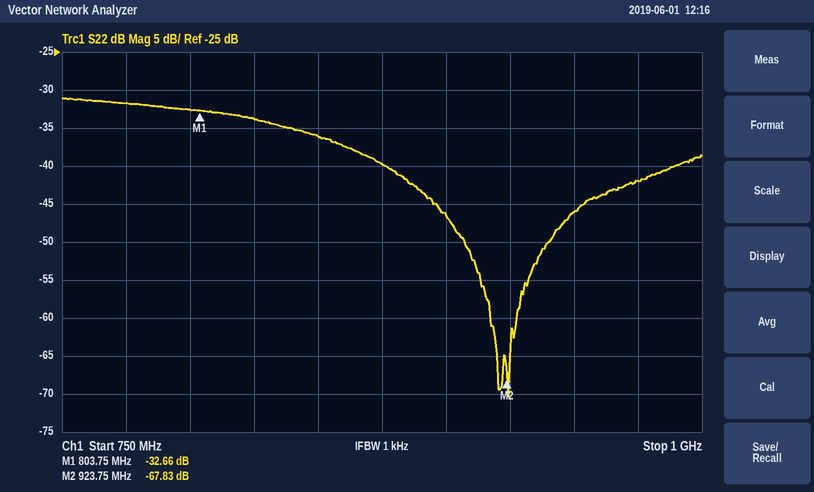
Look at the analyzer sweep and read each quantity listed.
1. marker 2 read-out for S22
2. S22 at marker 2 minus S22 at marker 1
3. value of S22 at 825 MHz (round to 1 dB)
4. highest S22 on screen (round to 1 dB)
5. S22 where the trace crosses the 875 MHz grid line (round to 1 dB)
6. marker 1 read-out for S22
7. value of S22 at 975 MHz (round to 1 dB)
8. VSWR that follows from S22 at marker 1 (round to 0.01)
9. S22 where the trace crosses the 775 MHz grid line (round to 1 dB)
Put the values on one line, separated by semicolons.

-67.83 dB; -35.17 dB; -34 dB; -31 dB; -40 dB; -32.66 dB; -42 dB; 1.05; -32 dB
